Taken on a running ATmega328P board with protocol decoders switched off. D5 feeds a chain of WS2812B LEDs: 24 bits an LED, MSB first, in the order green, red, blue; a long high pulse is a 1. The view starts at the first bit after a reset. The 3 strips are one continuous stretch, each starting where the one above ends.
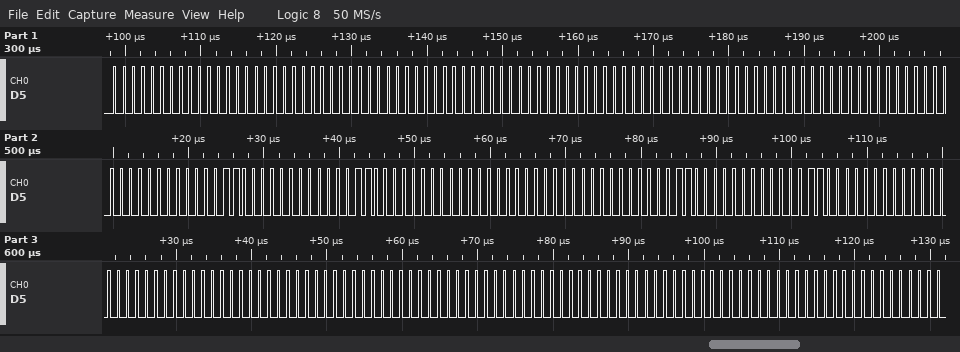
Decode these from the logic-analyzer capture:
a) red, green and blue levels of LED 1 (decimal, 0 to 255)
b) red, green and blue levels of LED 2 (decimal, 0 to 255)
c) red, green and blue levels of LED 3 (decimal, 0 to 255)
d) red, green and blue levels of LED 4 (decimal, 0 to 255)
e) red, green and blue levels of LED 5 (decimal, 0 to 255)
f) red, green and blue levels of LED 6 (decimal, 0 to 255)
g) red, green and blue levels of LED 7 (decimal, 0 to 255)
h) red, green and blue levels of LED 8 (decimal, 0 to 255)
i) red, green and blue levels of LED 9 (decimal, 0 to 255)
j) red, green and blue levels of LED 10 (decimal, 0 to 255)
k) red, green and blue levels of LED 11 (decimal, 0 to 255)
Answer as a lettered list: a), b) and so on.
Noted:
a) 0, 0, 0
b) 0, 0, 0
c) 0, 0, 0
d) 0, 0, 0
e) 0, 6, 24
f) 0, 0, 0
g) 0, 6, 24
h) 0, 0, 0
i) 0, 0, 0
j) 0, 0, 0
k) 0, 0, 0
